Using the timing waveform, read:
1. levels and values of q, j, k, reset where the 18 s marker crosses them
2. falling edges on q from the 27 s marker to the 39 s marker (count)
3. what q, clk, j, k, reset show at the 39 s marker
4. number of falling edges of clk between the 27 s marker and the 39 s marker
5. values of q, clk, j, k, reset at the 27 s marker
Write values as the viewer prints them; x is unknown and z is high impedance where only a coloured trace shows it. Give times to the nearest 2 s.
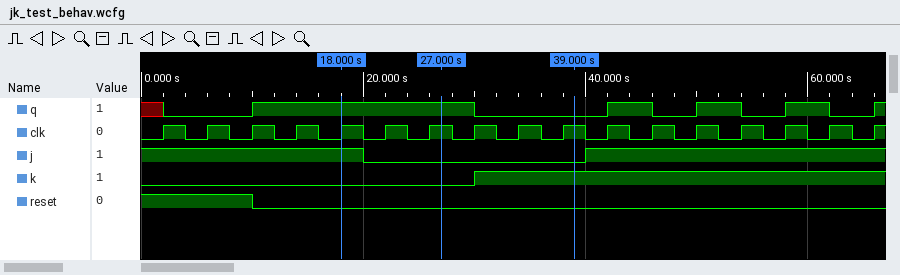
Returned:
q=1, j=1, k=0, reset=0
1
q=0, clk=1, j=0, k=1, reset=0
3
q=1, clk=1, j=0, k=0, reset=0
